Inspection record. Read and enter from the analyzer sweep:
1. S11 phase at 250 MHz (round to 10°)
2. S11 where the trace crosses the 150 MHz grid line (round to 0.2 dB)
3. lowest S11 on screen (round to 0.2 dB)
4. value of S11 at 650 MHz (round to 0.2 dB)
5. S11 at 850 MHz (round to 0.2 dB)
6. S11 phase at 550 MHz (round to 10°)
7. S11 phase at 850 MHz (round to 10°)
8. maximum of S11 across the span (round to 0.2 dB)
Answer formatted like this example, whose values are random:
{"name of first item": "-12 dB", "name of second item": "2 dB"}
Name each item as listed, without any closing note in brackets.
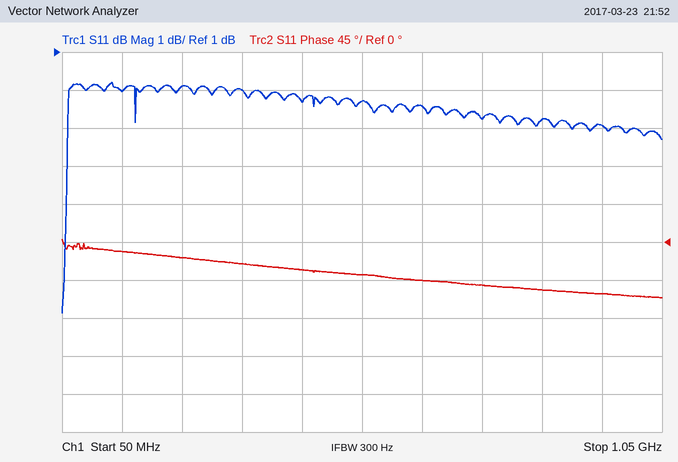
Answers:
{"S11 phase at 250 MHz": "-20°", "S11 where the trace crosses the 150 MHz grid line": "0.0 dB", "lowest S11 on screen": "-5.8 dB", "value of S11 at 650 MHz": "-0.4 dB", "S11 at 850 MHz": "-0.8 dB", "S11 phase at 550 MHz": "-40°", "S11 phase at 850 MHz": "-60°", "maximum of S11 across the span": "0.2 dB"}
